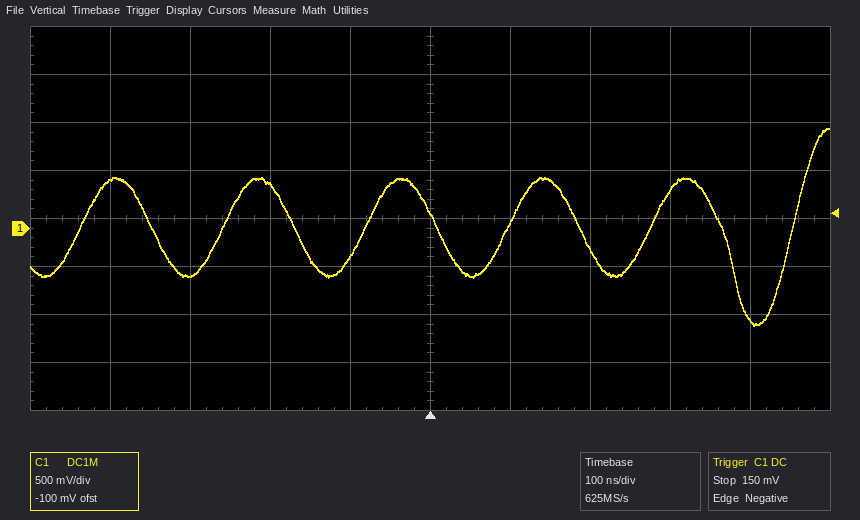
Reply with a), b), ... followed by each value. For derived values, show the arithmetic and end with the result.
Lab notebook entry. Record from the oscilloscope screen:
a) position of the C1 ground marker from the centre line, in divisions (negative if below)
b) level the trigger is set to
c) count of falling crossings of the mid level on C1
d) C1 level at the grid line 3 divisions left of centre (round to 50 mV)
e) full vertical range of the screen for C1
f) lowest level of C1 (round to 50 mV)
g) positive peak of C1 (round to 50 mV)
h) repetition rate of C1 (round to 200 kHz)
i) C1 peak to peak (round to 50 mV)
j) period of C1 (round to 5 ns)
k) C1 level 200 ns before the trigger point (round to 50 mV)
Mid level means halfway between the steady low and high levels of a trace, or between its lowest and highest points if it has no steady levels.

a) -0.2 div
b) 150 mV
c) 5
d) -500 mV
e) 4 V
f) -1.00 V
g) 1.05 V
h) 1 / 180 ns ≈ 5.6 MHz
i) 1.05 V − (-1.00 V) = 2.05 V
j) 180 ns
k) 450 mV
